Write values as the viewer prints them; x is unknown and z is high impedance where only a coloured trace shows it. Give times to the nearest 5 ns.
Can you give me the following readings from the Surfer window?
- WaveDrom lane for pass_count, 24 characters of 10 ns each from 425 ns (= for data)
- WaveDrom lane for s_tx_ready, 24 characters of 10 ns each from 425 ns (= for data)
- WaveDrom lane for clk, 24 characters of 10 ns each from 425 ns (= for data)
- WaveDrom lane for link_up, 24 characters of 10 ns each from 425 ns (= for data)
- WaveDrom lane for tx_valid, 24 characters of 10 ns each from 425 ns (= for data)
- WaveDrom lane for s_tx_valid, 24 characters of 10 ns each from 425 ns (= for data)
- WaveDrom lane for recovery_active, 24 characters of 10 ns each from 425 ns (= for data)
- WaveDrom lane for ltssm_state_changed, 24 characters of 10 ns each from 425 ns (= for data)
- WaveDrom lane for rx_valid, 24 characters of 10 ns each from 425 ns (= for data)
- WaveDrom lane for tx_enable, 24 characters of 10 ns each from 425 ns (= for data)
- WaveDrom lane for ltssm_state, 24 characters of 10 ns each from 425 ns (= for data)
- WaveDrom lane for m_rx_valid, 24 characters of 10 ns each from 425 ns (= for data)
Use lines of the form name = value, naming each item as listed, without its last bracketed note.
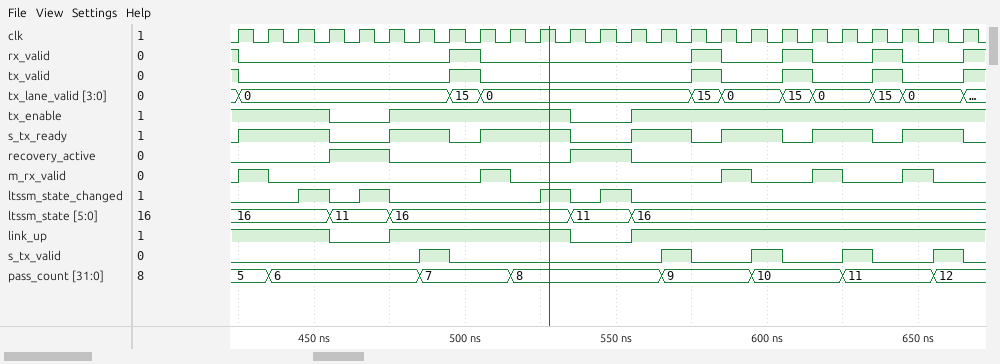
WaveDrom lane for pass_count, 24 characters of 10 ns each from 425 ns = {name: 'pass_count', wave: '==....=..=....=..=..=..=', data: '5 6 7 8 9 10 11 12'}
WaveDrom lane for s_tx_ready, 24 characters of 10 ns each from 425 ns = {name: 's_tx_ready', wave: '1..0.1.01..0.1.01.01.01.'}
WaveDrom lane for clk, 24 characters of 10 ns each from 425 ns = {name: 'clk', wave: 'p.......................'}
WaveDrom lane for link_up, 24 characters of 10 ns each from 425 ns = {name: 'link_up', wave: '1..0.1.....0.1..........'}
WaveDrom lane for tx_valid, 24 characters of 10 ns each from 425 ns = {name: 'tx_valid', wave: '0......10......10.10.10.'}
WaveDrom lane for s_tx_valid, 24 characters of 10 ns each from 425 ns = {name: 's_tx_valid', wave: '0.....10......10.10.10.1'}
WaveDrom lane for recovery_active, 24 characters of 10 ns each from 425 ns = {name: 'recovery_active', wave: '0..1.0.....1.0..........'}
WaveDrom lane for ltssm_state_changed, 24 characters of 10 ns each from 425 ns = {name: 'ltssm_state_changed', wave: '0.1010....1010..........'}
WaveDrom lane for rx_valid, 24 characters of 10 ns each from 425 ns = {name: 'rx_valid', wave: '0......10......10.10.10.'}
WaveDrom lane for tx_enable, 24 characters of 10 ns each from 425 ns = {name: 'tx_enable', wave: '1..0.1.....0.1..........'}
WaveDrom lane for ltssm_state, 24 characters of 10 ns each from 425 ns = {name: 'ltssm_state', wave: '=..=.=.....=.=..........', data: '16 11 16 11 16'}
WaveDrom lane for m_rx_valid, 24 characters of 10 ns each from 425 ns = {name: 'm_rx_valid', wave: '10......10......10.10.10'}
